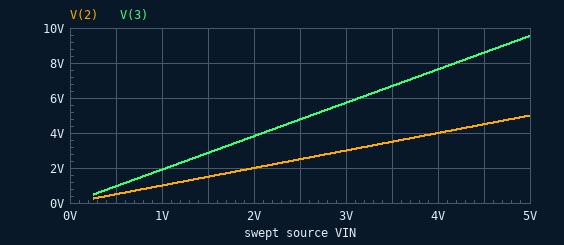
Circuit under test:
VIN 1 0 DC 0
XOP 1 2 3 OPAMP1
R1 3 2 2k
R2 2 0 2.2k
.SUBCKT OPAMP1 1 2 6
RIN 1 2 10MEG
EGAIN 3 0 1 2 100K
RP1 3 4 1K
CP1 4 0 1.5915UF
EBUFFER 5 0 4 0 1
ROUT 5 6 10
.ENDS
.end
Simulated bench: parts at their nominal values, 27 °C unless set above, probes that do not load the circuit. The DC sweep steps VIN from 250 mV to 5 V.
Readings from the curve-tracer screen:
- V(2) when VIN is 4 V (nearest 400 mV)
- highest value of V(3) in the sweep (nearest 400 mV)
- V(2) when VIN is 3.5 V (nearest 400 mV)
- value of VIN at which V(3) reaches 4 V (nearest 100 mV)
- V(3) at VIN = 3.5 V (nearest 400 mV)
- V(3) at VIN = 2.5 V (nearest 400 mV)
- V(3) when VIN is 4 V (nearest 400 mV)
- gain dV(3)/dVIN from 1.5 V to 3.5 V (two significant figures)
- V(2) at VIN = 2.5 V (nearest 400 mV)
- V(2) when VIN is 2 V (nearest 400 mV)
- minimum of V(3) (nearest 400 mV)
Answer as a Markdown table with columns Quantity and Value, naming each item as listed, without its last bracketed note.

| Quantity | Value |
|---|---|
| V(2) when VIN is 4 V | 4.0 V |
| highest value of V(3) in the sweep | 9.6 V |
| V(2) when VIN is 3.5 V | 3.6 V |
| value of VIN at which V(3) reaches 4 V | 2.1 V |
| V(3) at VIN = 3.5 V | 6.8 V |
| V(3) at VIN = 2.5 V | 4.8 V |
| V(3) when VIN is 4 V | 7.6 V |
| gain dV(3)/dVIN from 1.5 V to 3.5 V | 1.9 V/V |
| V(2) at VIN = 2.5 V | 2.4 V |
| V(2) when VIN is 2 V | 2.0 V |
| minimum of V(3) | 400 mV |
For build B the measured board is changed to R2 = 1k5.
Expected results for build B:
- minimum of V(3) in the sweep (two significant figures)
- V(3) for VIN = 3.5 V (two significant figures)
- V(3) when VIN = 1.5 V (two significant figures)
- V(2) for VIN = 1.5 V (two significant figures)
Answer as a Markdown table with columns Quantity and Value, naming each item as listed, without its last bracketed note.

| Quantity | Value |
|---|---|
| minimum of V(3) in the sweep | 580 mV |
| V(3) for VIN = 3.5 V | 8.2 V |
| V(3) when VIN = 1.5 V | 3.5 V |
| V(2) for VIN = 1.5 V | 1.5 V |
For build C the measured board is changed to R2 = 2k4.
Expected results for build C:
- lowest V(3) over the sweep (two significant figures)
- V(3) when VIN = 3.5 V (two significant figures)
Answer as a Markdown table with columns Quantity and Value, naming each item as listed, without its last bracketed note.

| Quantity | Value |
|---|---|
| lowest V(3) over the sweep | 460 mV |
| V(3) when VIN = 3.5 V | 6.4 V |
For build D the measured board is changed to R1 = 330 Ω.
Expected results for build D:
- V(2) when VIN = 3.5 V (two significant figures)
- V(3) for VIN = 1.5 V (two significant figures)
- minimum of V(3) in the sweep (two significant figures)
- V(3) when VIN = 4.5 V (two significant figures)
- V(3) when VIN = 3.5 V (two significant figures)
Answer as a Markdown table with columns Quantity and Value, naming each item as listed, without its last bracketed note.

| Quantity | Value |
|---|---|
| V(2) when VIN = 3.5 V | 3.5 V |
| V(3) for VIN = 1.5 V | 1.7 V |
| minimum of V(3) in the sweep | 290 mV |
| V(3) when VIN = 4.5 V | 5.2 V |
| V(3) when VIN = 3.5 V | 4.0 V |
